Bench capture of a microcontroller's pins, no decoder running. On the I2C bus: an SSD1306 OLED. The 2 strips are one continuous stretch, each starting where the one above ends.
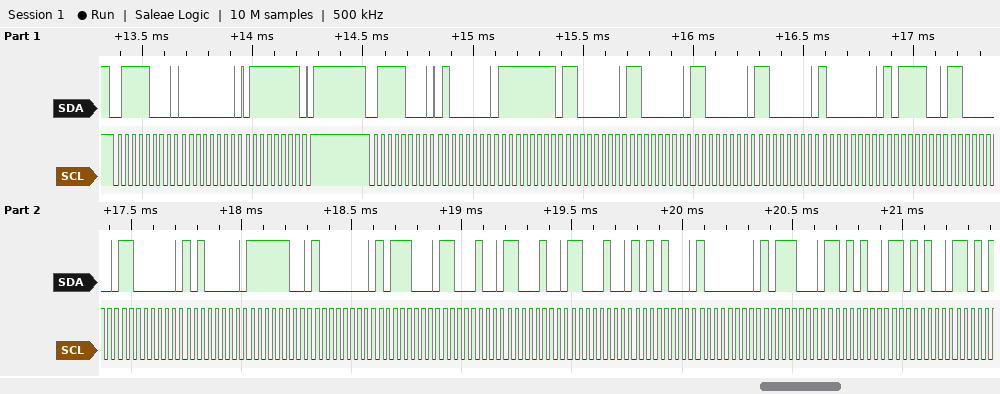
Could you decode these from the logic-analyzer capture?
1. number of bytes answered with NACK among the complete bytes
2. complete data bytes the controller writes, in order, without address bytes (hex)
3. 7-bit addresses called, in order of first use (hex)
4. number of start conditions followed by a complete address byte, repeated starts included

0
00 7F 40 FF C0 C0 C0 C0 80 BC C0 C0 A0 FC 80 B8 C4 C4 C4 A8 80 B8 D4 D4
0x3C
2
